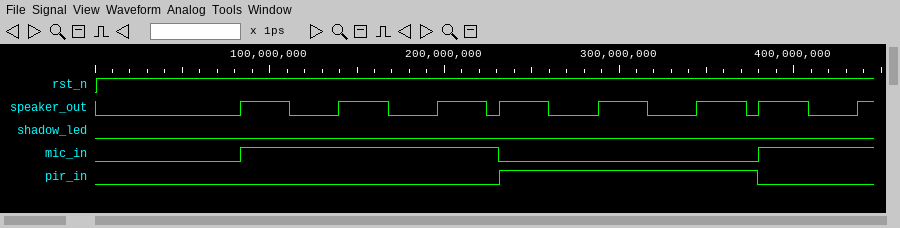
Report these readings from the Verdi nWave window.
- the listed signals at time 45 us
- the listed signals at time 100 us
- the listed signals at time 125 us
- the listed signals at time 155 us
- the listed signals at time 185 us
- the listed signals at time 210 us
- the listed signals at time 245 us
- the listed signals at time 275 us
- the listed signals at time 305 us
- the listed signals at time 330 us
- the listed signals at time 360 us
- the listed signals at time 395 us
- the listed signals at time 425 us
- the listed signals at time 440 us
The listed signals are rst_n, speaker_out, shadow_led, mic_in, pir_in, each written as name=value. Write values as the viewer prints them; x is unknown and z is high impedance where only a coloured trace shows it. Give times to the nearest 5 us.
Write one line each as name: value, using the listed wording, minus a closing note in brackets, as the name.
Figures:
the listed signals at time 45 us: rst_n=1, speaker_out=0, shadow_led=0, mic_in=0, pir_in=0
the listed signals at time 100 us: rst_n=1, speaker_out=1, shadow_led=0, mic_in=1, pir_in=0
the listed signals at time 125 us: rst_n=1, speaker_out=0, shadow_led=0, mic_in=1, pir_in=0
the listed signals at time 155 us: rst_n=1, speaker_out=1, shadow_led=0, mic_in=1, pir_in=0
the listed signals at time 185 us: rst_n=1, speaker_out=0, shadow_led=0, mic_in=1, pir_in=0
the listed signals at time 210 us: rst_n=1, speaker_out=1, shadow_led=0, mic_in=1, pir_in=0
the listed signals at time 245 us: rst_n=1, speaker_out=1, shadow_led=0, mic_in=0, pir_in=1
the listed signals at time 275 us: rst_n=1, speaker_out=0, shadow_led=0, mic_in=0, pir_in=1
the listed signals at time 305 us: rst_n=1, speaker_out=1, shadow_led=0, mic_in=0, pir_in=1
the listed signals at time 330 us: rst_n=1, speaker_out=0, shadow_led=0, mic_in=0, pir_in=1
the listed signals at time 360 us: rst_n=1, speaker_out=1, shadow_led=0, mic_in=0, pir_in=1
the listed signals at time 395 us: rst_n=1, speaker_out=1, shadow_led=0, mic_in=1, pir_in=0
the listed signals at time 425 us: rst_n=1, speaker_out=0, shadow_led=0, mic_in=1, pir_in=0
the listed signals at time 440 us: rst_n=1, speaker_out=1, shadow_led=0, mic_in=1, pir_in=0
